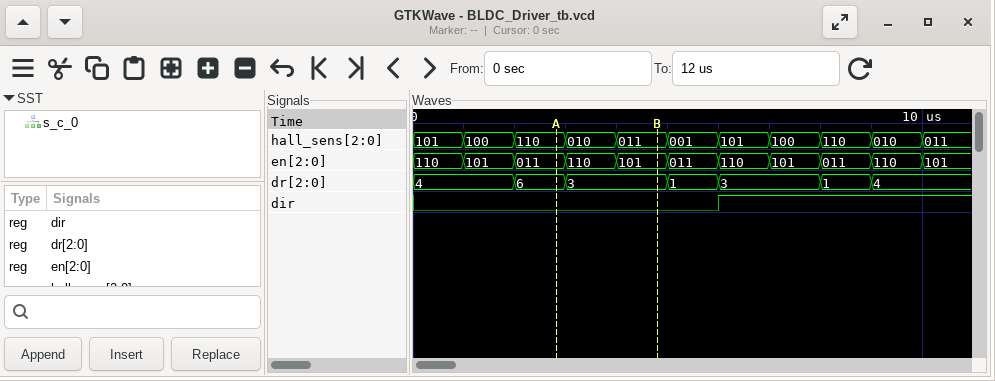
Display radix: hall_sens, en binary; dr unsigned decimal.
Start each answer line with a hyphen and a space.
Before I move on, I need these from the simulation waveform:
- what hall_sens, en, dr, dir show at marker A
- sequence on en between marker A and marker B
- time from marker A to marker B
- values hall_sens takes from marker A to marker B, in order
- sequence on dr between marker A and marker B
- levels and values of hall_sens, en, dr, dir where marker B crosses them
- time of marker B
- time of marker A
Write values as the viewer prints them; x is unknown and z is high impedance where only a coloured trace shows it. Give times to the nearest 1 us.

- hall_sens=110, en=011, dr=6, dir=0
- 011, 110, 101
- 2 us
- 110, 010, 011
- 6, 3
- hall_sens=011, en=101, dr=3, dir=0
- 5 us
- 3 us
